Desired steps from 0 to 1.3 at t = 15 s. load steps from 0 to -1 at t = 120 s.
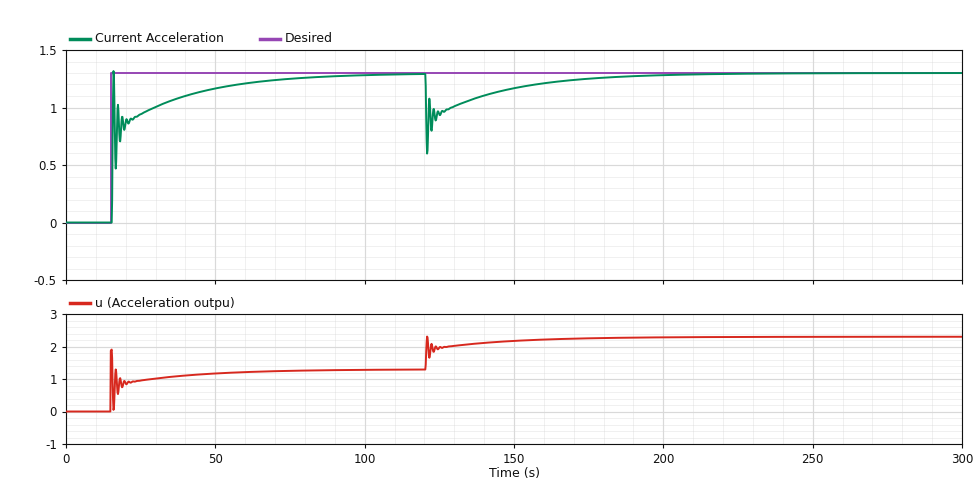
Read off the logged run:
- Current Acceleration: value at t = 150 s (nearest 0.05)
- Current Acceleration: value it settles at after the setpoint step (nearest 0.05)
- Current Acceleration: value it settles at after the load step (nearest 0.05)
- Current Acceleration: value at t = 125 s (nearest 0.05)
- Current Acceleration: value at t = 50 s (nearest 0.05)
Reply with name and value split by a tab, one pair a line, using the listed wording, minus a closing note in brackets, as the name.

Current Acceleration: value at t = 150 s	1.15
Current Acceleration: value it settles at after the setpoint step	1.30
Current Acceleration: value it settles at after the load step	1.30
Current Acceleration: value at t = 125 s	0.95
Current Acceleration: value at t = 50 s	1.15
